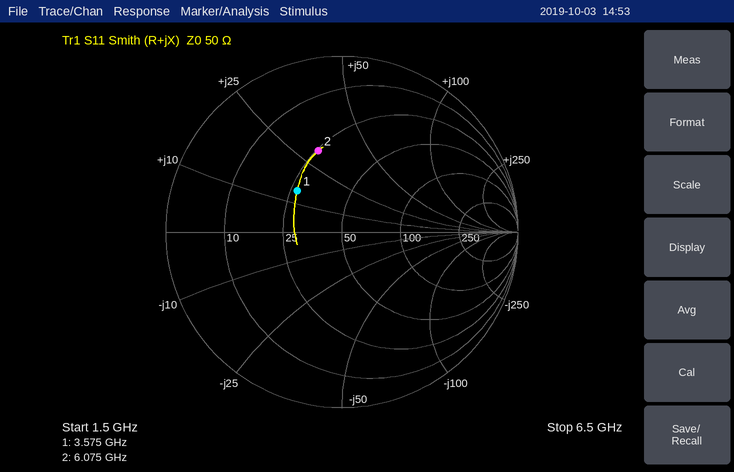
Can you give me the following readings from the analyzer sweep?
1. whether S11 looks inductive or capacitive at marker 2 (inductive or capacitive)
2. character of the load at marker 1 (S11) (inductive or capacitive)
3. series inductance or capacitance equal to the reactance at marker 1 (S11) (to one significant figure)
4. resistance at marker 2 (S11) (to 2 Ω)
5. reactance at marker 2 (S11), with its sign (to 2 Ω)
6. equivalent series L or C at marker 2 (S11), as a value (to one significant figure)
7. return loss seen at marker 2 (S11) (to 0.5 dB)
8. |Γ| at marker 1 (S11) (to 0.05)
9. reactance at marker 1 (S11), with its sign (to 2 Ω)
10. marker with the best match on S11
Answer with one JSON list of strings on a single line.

["inductive", "inductive", "600 pH", "26 Ω", "+30 Ω", "800 pH", "6.5 dB", "0.35", "+14 Ω", "marker 1"]
